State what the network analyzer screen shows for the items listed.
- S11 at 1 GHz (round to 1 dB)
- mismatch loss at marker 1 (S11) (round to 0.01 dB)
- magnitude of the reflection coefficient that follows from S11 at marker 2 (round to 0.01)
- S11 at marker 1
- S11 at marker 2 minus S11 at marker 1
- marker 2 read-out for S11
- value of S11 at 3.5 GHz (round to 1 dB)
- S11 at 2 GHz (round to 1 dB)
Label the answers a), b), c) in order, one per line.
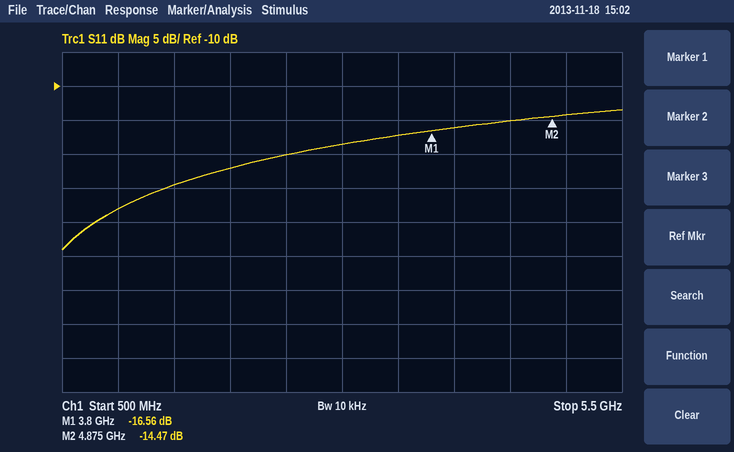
a) -28 dB
b) 0.10 dB
c) 0.19
d) -16.56 dB
e) 2.09 dB
f) -14.47 dB
g) -17 dB
h) -22 dB
